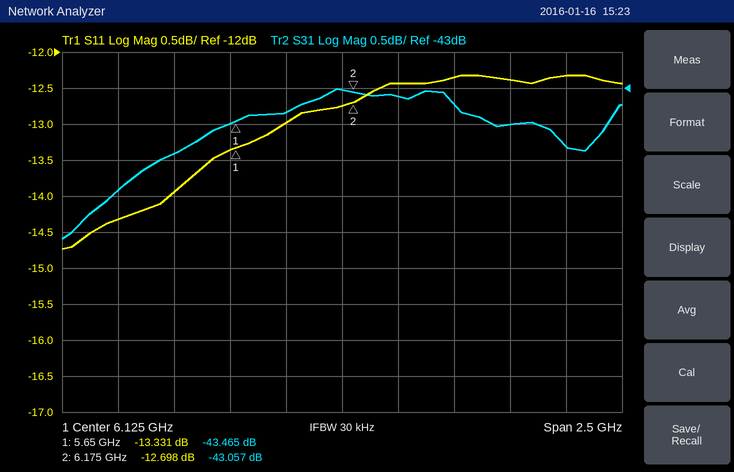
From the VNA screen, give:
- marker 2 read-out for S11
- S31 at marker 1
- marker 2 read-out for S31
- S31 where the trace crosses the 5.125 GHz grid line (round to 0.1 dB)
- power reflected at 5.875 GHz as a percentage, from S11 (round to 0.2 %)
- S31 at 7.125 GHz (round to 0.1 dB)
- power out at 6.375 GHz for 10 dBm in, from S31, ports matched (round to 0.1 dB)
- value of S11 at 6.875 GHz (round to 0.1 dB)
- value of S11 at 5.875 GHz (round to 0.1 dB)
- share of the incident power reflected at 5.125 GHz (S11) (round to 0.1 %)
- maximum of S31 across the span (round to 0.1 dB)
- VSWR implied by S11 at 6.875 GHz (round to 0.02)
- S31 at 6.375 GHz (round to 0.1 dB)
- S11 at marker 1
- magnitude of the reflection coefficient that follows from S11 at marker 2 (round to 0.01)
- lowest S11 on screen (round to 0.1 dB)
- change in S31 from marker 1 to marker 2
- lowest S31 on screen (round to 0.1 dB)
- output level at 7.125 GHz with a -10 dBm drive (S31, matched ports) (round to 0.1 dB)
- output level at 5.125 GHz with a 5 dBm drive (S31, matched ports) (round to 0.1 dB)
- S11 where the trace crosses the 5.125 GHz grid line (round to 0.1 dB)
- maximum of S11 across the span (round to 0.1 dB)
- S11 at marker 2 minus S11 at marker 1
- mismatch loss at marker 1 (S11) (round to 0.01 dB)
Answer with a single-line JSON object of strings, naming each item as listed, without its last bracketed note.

{"marker 2 read-out for S11": "-12.698 dB", "S31 at marker 1": "-43.465 dB", "marker 2 read-out for S31": "-43.057 dB", "S31 where the trace crosses the 5.125 GHz grid line": "-44.4 dB", "power reflected at 5.875 GHz as a percentage, from S11": "5.0 %", "S31 at 7.125 GHz": "-43.8 dB", "power out at 6.375 GHz for 10 dBm in, from S31, ports matched": "-33.1 dBm", "value of S11 at 6.875 GHz": "-12.4 dB", "value of S11 at 5.875 GHz": "-13.0 dB", "share of the incident power reflected at 5.125 GHz (S11)": "3.7 %", "maximum of S31 across the span": "-43.0 dB", "VSWR implied by S11 at 6.875 GHz": "1.64", "S31 at 6.375 GHz": "-43.1 dB", "S11 at marker 1": "-13.331 dB", "magnitude of the reflection coefficient that follows from S11 at marker 2": "0.23", "lowest S11 on screen": "-14.7 dB", "change in S31 from marker 1 to marker 2": "0.408 dB", "lowest S31 on screen": "-45.1 dB", "output level at 7.125 GHz with a -10 dBm drive (S31, matched ports)": "-53.8 dBm", "output level at 5.125 GHz with a 5 dBm drive (S31, matched ports)": "-39.4 dBm", "S11 where the trace crosses the 5.125 GHz grid line": "-14.3 dB", "maximum of S11 across the span": "-12.3 dB", "S11 at marker 2 minus S11 at marker 1": "0.633 dB", "mismatch loss at marker 1 (S11)": "0.21 dB"}
